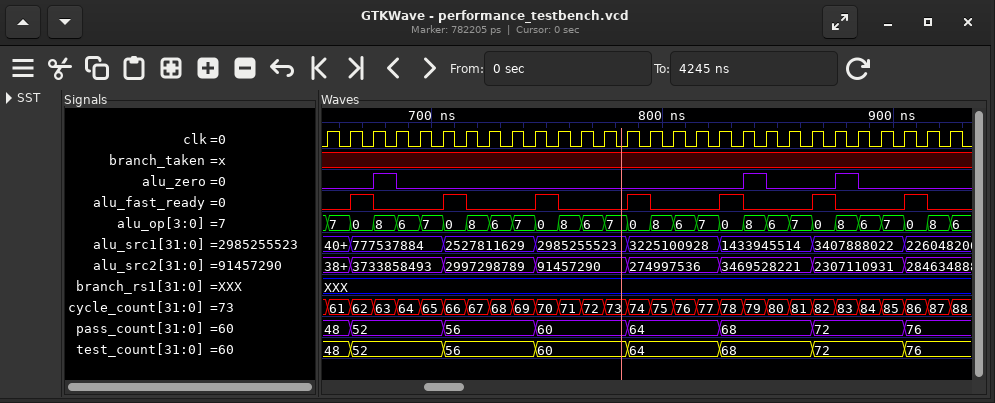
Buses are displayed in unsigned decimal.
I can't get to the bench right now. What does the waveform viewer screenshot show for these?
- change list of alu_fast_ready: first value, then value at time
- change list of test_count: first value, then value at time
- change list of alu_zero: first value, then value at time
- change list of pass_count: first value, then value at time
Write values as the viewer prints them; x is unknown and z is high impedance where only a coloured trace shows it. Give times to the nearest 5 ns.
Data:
0, 1 at 665 ns, 0 at 675 ns, 1 at 705 ns, 0 at 715 ns, 1 at 745 ns, 0 at 755 ns, 1 at 785 ns, 0 at 795 ns, 1 at 825 ns, 0 at 835 ns, 1 at 865 ns, 0 at 875 ns, 1 at 905 ns, 0 at 915 ns
48, 52 at 665 ns, 56 at 705 ns, 60 at 745 ns, 64 at 785 ns, 68 at 825 ns, 72 at 865 ns, 76 at 905 ns
0, 1 at 675 ns, 0 at 685 ns, 1 at 835 ns, 0 at 845 ns, 1 at 875 ns, 0 at 885 ns
48, 52 at 665 ns, 56 at 705 ns, 60 at 745 ns, 64 at 785 ns, 68 at 825 ns, 72 at 865 ns, 76 at 905 ns
